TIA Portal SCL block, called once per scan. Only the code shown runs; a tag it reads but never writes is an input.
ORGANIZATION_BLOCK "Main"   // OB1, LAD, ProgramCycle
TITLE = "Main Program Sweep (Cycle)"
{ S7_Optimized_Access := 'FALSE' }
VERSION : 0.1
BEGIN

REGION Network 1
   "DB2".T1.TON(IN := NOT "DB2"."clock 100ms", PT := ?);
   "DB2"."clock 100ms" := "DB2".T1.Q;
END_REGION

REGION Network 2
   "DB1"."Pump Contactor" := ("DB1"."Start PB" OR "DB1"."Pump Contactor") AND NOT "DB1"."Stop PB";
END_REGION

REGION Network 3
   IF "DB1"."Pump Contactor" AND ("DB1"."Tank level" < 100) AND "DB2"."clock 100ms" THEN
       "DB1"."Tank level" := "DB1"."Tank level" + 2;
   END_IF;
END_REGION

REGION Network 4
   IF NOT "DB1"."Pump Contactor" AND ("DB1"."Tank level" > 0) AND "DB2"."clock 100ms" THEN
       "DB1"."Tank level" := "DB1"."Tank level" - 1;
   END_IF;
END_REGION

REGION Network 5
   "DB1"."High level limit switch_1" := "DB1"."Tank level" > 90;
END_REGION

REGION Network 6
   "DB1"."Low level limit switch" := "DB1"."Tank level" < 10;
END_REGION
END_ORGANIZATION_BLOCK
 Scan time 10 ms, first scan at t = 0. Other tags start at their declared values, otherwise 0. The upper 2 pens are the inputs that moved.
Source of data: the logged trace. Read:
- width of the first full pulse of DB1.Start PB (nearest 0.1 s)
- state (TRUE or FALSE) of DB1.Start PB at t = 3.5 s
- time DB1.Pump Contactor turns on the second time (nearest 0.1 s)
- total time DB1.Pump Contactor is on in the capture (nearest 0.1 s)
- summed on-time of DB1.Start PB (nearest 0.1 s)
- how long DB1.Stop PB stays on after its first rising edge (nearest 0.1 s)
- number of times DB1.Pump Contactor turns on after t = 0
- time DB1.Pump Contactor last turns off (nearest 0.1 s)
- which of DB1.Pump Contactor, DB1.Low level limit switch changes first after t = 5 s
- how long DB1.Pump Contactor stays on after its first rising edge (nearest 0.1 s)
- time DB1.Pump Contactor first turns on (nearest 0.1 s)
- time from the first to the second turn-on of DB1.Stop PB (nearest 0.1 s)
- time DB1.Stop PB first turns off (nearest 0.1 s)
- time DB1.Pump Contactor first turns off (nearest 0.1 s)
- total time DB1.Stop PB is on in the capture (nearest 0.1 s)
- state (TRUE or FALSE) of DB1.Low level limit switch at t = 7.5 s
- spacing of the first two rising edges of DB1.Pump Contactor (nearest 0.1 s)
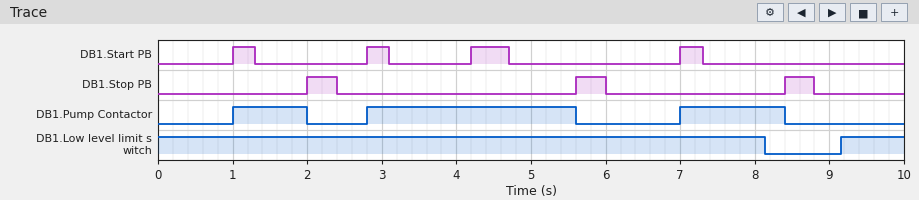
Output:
0.3 s
FALSE
2.8 s
5.2 s
1.4 s
0.4 s
3
8.4 s
DB1.Pump Contactor
1.0 s
1.0 s
3.6 s
2.4 s
2.0 s
1.2 s
TRUE
1.8 s
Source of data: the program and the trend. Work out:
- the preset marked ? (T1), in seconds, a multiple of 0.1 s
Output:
1.0 s
